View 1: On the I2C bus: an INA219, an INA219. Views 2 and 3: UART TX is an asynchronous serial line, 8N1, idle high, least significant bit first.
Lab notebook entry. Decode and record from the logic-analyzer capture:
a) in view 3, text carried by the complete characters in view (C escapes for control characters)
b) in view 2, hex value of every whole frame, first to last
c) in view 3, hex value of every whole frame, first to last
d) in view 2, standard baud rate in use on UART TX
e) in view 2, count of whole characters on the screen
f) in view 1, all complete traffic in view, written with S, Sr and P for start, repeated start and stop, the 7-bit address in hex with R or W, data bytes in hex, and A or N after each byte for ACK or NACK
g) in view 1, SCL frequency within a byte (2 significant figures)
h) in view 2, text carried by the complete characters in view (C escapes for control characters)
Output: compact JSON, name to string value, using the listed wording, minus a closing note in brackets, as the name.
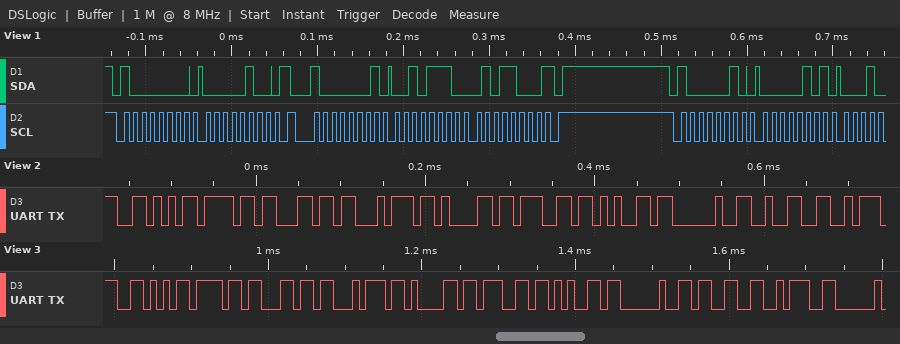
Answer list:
{"in view 3, text carried by the complete characters in view": "\"Voltage 3:\"", "in view 2, hex value of every whole frame, first to last": "56 6F 6C 74 61 67 65 20 32", "in view 3, hex value of every whole frame, first to last": "56 6F 6C 74 61 67 65 20 33 3A", "in view 2, standard baud rate in use on UART TX": "115200 baud", "in view 2, count of whole characters on the screen": "9", "in view 1, all complete traffic in view, written with S, Sr and P for start, repeated start and stop, the 7-bit address in hex with R or W, data bytes in hex, and A or N after each byte for ACK or NACK": "S 40W A 04 A Sr 40R A 2E A 58 N P S 41W A 05 A", "in view 1, SCL frequency within a byte": "100 kHz", "in view 2, text carried by the complete characters in view": "\"Voltage 2\""}
